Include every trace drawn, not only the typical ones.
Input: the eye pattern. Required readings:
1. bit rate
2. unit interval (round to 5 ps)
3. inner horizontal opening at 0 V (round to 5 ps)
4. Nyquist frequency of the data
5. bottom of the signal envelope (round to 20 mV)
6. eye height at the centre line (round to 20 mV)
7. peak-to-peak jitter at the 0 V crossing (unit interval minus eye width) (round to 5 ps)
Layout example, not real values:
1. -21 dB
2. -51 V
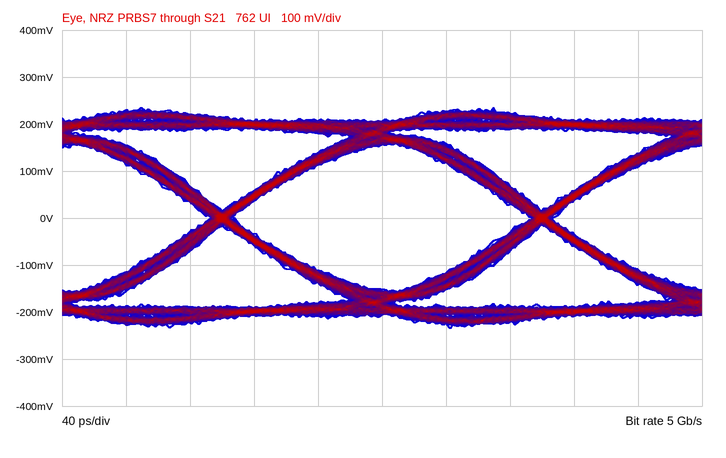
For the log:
1. 5 Gb/s
2. 200 ps
3. 185 ps
4. 2.5 GHz
5. -240 mV
6. 300 mV
7. 15 ps
